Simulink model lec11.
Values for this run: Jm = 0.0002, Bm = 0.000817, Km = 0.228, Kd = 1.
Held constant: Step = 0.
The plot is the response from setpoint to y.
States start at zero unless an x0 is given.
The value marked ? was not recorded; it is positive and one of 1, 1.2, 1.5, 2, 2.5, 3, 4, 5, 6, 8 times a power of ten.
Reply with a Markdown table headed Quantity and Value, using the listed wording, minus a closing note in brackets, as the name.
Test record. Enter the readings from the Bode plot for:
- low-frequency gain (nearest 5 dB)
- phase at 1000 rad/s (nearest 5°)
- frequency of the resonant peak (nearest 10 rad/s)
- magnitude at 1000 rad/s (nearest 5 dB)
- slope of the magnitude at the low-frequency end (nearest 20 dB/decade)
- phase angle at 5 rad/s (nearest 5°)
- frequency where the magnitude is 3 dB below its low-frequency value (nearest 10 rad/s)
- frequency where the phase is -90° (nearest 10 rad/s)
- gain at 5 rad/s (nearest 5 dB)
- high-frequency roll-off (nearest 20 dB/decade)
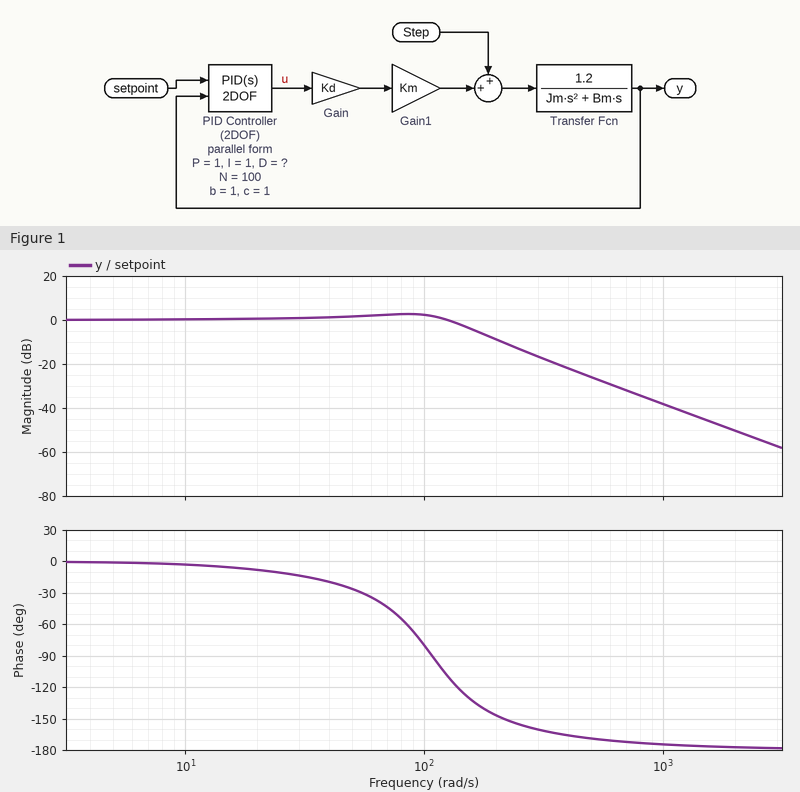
| Quantity | Value |
|---|---|
| low-frequency gain | 0 dB |
| phase at 1000 rad/s | -175° |
| frequency of the resonant peak | 80 rad/s |
| magnitude at 1000 rad/s | -40 dB |
| slope of the magnitude at the low-frequency end | 0 dB/decade |
| phase angle at 5 rad/s | 0° |
| frequency where the magnitude is 3 dB below its low-frequency value | 150 rad/s |
| frequency where the phase is -90° | 110 rad/s |
| gain at 5 rad/s | 0 dB |
| high-frequency roll-off | -40 dB/decade |
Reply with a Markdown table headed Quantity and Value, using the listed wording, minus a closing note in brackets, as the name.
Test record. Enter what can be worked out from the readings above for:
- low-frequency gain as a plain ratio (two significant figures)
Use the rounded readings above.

| Quantity | Value |
|---|---|
| low-frequency gain as a plain ratio | 1.0 |
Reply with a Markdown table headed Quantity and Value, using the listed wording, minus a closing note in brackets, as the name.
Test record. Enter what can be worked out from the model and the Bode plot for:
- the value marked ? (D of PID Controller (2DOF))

| Quantity | Value |
|---|---|
| the value marked ? (D of PID Controller (2DOF)) | 0.08 |
